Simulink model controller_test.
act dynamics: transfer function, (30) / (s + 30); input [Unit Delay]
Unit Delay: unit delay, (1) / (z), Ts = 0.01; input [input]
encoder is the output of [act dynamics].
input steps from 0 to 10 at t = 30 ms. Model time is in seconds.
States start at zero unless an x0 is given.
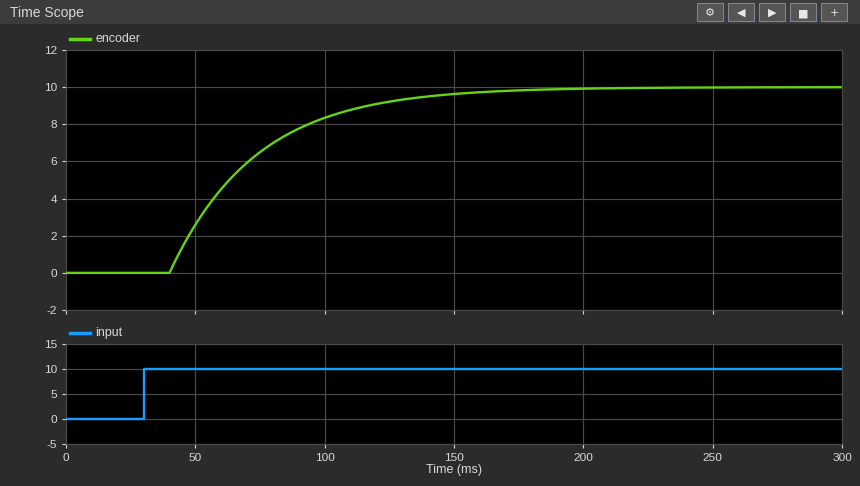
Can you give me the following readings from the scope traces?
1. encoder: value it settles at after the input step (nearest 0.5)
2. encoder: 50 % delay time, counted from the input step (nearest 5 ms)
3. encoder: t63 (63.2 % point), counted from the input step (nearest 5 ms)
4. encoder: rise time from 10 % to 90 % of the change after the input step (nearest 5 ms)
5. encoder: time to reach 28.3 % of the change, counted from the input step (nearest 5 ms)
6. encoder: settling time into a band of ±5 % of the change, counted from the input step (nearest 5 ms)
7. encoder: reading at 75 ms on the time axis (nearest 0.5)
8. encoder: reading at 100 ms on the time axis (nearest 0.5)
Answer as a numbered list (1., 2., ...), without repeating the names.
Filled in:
1. 10.0
2. 35 ms
3. 45 ms
4. 75 ms
5. 20 ms
6. 110 ms
7. 6.5
8. 8.5
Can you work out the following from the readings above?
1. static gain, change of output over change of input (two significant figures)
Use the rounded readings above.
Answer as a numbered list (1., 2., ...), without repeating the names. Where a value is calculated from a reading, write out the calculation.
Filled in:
1. (10 - 0) / (10 - 0) = 1.0
